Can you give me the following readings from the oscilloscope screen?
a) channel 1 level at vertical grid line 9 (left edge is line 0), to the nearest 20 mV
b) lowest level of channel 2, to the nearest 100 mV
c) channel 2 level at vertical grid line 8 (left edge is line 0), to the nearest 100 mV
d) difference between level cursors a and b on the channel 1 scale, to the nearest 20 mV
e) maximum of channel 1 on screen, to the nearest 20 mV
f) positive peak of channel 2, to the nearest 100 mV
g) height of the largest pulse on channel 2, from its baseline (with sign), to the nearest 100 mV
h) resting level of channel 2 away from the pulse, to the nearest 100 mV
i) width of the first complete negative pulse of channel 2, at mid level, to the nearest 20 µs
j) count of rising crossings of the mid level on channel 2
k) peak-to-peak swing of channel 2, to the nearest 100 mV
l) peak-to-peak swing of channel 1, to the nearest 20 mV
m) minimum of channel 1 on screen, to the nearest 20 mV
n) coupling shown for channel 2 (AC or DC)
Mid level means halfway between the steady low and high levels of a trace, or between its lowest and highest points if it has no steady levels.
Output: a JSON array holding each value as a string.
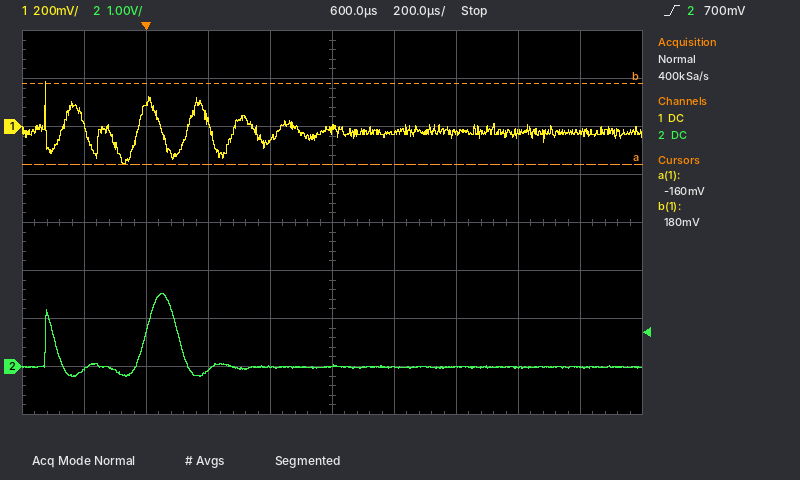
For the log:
["-20 mV", "-200 mV", "0.0 V", "340 mV", "180 mV", "1.5 V", "+1.5 V", "0.0 V", "300 µs", "2", "1.7 V", "340 mV", "-160 mV", "DC"]
